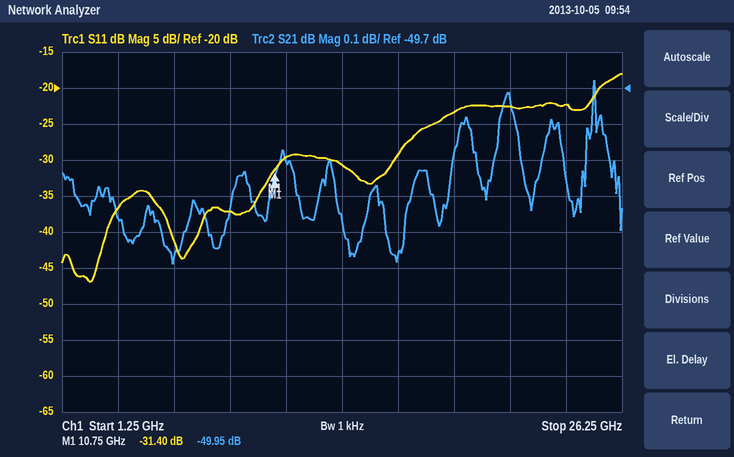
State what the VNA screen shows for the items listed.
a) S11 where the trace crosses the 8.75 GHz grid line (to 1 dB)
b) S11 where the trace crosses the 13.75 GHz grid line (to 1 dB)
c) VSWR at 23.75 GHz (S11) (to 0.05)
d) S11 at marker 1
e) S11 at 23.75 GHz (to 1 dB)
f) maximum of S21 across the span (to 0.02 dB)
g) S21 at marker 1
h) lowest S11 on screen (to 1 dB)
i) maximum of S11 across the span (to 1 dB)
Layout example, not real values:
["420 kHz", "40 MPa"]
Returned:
["-37 dB", "-31 dB", "1.15", "-31.40 dB", "-22 dB", "-49.68 dB", "-49.95 dB", "-47 dB", "-18 dB"]
